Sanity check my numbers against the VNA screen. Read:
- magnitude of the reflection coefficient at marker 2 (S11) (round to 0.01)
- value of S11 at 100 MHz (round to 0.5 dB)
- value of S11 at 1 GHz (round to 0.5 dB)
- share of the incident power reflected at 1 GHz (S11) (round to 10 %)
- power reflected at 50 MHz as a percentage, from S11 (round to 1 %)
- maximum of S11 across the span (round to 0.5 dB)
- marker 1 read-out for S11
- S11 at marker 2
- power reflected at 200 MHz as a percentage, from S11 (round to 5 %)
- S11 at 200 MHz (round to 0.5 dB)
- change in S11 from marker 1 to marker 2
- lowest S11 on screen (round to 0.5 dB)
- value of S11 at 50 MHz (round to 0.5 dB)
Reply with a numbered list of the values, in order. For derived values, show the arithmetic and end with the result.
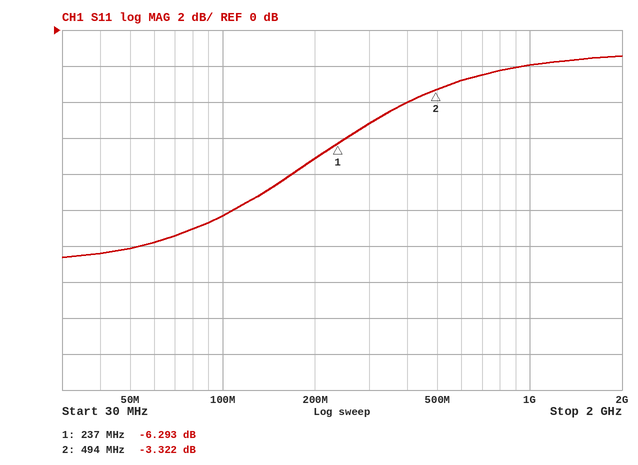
1. 10^(-3.322/20) ≈ 0.68
2. -10.5 dB
3. -2.0 dB
4. 10^(-2/10) ≈ 63.1 %, so 60 % to the nearest 10 %
5. 10^(-12/10) ≈ 6 %
6. -1.5 dB
7. -6.293 dB
8. -3.322 dB
9. 10^(-7/10) ≈ 20 %
10. -7.0 dB
11. -3.322 − (-6.293) = 2.971 dB
12. -12.5 dB
13. -12.0 dB
